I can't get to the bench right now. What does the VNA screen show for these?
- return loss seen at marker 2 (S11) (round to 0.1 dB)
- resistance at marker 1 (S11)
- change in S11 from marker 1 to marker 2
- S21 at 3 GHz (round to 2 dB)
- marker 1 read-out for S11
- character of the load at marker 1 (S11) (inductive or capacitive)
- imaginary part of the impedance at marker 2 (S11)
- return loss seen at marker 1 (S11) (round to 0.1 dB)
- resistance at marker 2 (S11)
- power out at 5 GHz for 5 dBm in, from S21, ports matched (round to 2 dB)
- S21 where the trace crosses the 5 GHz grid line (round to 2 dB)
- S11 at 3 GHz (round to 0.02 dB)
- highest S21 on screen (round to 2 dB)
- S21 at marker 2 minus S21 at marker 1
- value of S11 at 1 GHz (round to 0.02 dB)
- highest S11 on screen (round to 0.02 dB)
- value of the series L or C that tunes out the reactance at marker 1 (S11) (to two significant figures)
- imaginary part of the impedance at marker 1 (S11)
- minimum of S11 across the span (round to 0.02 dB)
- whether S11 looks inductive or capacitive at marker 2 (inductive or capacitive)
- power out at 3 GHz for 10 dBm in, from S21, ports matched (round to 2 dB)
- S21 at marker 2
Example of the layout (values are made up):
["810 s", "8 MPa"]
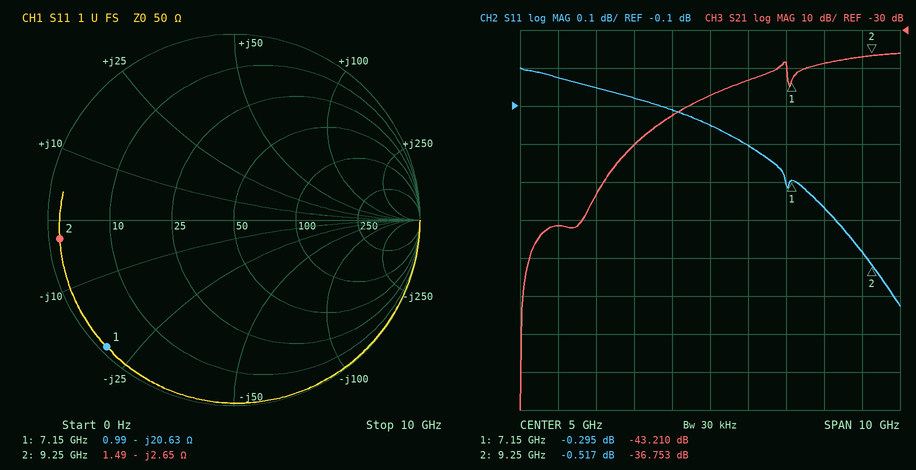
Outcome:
["0.5 dB", "0.99 Ω", "-0.222 dB", "-60 dB", "-0.295 dB", "capacitive", "-2.65 Ω", "0.3 dB", "1.49 Ω", "-42 dBm", "-48 dB", "-0.08 dB", "-36 dB", "6.457 dB", "-0.02 dB", "0.00 dB", "460 pH", "-20.63 Ω", "-0.62 dB", "capacitive", "-50 dBm", "-36.753 dB"]
